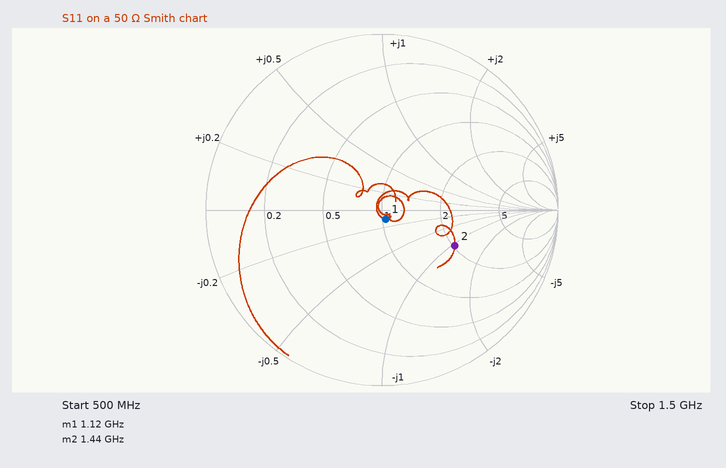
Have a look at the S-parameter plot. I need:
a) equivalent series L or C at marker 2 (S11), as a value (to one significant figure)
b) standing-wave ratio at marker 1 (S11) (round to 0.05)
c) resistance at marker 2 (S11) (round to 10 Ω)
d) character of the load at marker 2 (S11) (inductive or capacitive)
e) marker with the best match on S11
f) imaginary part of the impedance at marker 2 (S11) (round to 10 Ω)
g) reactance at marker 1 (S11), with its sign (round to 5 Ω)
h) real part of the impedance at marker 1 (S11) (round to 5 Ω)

2 pF
1.10
100 Ω
capacitive
marker 1
-50 Ω
-5 Ω
50 Ω
